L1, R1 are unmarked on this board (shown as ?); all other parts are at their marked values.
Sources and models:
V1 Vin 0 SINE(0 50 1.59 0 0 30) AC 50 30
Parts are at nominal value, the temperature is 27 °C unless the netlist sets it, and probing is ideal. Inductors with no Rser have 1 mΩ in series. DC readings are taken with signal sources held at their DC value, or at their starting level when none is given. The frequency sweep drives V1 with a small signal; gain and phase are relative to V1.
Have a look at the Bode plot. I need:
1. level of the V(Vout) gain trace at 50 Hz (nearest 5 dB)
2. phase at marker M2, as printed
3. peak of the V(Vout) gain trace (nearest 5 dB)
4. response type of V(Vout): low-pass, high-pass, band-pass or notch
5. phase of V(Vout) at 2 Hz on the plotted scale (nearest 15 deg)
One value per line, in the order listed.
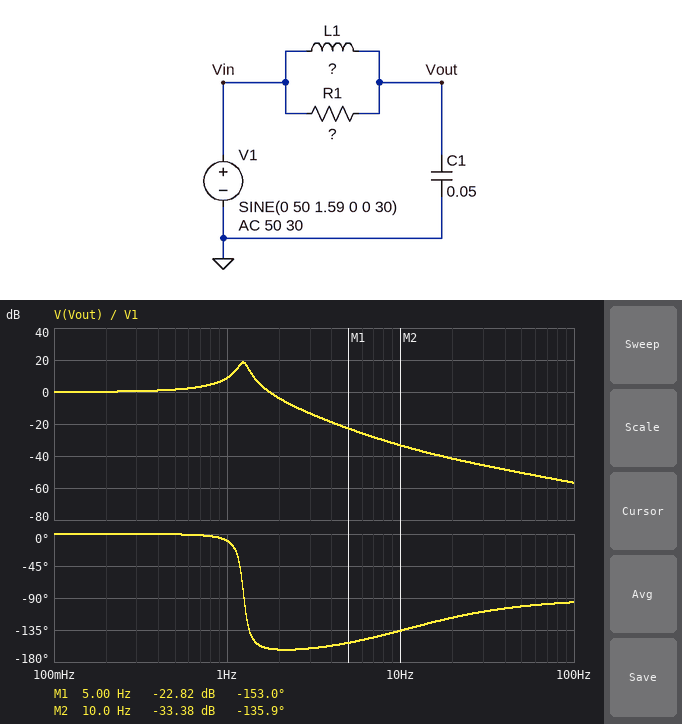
-50 dB
-135.9 deg
20 dB
low-pass
-165 deg
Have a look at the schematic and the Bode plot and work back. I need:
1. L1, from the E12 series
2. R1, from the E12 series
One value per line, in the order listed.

330 mH
22 Ω
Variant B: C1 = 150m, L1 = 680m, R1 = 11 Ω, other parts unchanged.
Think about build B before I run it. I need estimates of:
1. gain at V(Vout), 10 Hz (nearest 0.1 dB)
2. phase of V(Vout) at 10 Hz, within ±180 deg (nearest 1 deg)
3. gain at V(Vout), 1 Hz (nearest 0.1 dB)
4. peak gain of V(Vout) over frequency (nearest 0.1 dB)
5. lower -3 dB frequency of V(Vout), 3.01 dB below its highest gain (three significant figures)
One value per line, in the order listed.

-40.0 dB
-104 deg
-9.1 dB
14.4 dB
443 mHz
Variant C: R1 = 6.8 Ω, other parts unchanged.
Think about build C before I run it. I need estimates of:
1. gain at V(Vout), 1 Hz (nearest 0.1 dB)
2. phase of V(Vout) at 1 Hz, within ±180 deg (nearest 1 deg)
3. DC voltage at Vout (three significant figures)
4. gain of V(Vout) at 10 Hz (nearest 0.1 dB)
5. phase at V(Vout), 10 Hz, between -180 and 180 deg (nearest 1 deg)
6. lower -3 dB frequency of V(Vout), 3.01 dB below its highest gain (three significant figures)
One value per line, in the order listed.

7.1 dB
-24 deg
25.0 V
-26.0 dB
-105 deg
939 mHz
